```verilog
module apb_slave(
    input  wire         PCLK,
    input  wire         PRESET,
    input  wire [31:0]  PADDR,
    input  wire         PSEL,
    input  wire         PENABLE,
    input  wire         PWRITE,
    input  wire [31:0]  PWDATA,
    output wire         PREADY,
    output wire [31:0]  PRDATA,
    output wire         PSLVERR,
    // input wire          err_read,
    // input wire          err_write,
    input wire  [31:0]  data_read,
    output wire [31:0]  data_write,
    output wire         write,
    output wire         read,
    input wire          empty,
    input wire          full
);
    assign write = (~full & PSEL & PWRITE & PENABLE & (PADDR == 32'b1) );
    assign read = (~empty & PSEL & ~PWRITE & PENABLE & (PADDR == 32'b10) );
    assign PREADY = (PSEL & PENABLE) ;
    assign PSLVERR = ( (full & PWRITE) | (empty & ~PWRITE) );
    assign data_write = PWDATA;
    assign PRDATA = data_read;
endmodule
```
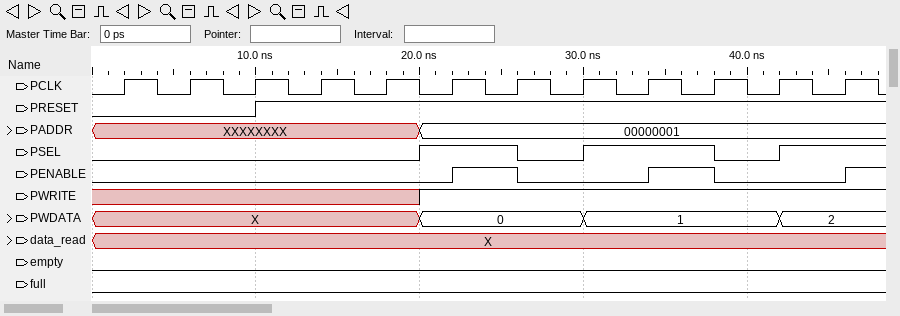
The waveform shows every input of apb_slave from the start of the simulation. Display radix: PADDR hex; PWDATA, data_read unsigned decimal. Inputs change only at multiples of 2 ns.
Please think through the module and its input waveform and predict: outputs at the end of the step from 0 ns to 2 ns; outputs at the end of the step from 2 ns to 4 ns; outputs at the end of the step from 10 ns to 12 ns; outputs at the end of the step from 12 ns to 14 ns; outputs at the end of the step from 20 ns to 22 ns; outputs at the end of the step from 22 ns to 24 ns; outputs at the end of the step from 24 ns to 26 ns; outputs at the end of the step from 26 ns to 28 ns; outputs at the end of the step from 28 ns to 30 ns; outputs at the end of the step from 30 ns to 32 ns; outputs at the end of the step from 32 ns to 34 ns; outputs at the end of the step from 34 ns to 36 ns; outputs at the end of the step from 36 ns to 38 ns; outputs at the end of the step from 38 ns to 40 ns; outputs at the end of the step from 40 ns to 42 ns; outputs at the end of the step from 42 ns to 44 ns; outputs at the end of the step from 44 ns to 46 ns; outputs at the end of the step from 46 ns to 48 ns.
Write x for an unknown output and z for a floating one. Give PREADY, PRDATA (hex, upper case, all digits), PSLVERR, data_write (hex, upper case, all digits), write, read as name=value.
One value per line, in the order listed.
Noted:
PREADY=0, PRDATA=x, PSLVERR=0, data_write=x, write=0, read=0
PREADY=0, PRDATA=x, PSLVERR=0, data_write=x, write=0, read=0
PREADY=0, PRDATA=x, PSLVERR=0, data_write=x, write=0, read=0
PREADY=0, PRDATA=x, PSLVERR=0, data_write=x, write=0, read=0
PREADY=0, PRDATA=x, PSLVERR=0, data_write=00000000, write=0, read=0
PREADY=1, PRDATA=x, PSLVERR=0, data_write=00000000, write=1, read=0
PREADY=1, PRDATA=x, PSLVERR=0, data_write=00000000, write=1, read=0
PREADY=0, PRDATA=x, PSLVERR=0, data_write=00000000, write=0, read=0
PREADY=0, PRDATA=x, PSLVERR=0, data_write=00000000, write=0, read=0
PREADY=0, PRDATA=x, PSLVERR=0, data_write=00000001, write=0, read=0
PREADY=0, PRDATA=x, PSLVERR=0, data_write=00000001, write=0, read=0
PREADY=1, PRDATA=x, PSLVERR=0, data_write=00000001, write=1, read=0
PREADY=1, PRDATA=x, PSLVERR=0, data_write=00000001, write=1, read=0
PREADY=0, PRDATA=x, PSLVERR=0, data_write=00000001, write=0, read=0
PREADY=0, PRDATA=x, PSLVERR=0, data_write=00000001, write=0, read=0
PREADY=0, PRDATA=x, PSLVERR=0, data_write=00000002, write=0, read=0
PREADY=0, PRDATA=x, PSLVERR=0, data_write=00000002, write=0, read=0
PREADY=1, PRDATA=x, PSLVERR=0, data_write=00000002, write=1, read=0
